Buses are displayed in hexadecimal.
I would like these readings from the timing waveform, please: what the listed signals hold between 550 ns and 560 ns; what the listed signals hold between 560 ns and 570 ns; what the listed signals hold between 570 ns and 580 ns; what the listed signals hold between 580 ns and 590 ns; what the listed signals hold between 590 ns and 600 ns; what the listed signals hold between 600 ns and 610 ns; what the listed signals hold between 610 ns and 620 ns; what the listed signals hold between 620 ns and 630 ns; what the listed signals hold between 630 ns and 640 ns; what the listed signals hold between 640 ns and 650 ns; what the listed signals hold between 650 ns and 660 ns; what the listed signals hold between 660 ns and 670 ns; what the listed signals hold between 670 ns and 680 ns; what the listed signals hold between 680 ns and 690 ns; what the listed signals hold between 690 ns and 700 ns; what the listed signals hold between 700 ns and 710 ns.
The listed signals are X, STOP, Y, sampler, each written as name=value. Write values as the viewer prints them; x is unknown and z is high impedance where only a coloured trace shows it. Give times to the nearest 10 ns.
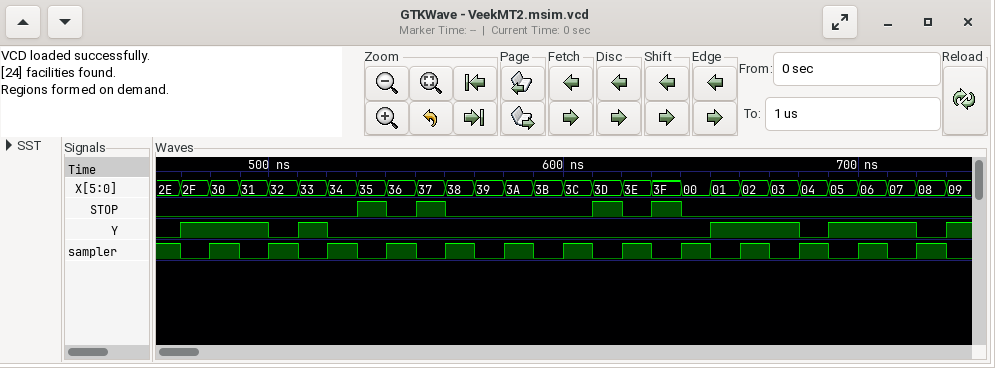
X=37, STOP=1, Y=0, sampler=0
X=38, STOP=0, Y=0, sampler=1
X=39, STOP=0, Y=0, sampler=0
X=3A, STOP=0, Y=0, sampler=1
X=3B, STOP=0, Y=0, sampler=0
X=3C, STOP=0, Y=0, sampler=1
X=3D, STOP=1, Y=0, sampler=0
X=3E, STOP=0, Y=0, sampler=1
X=3F, STOP=1, Y=0, sampler=0
X=00, STOP=0, Y=0, sampler=1
X=01, STOP=0, Y=1, sampler=0
X=02, STOP=0, Y=1, sampler=1
X=03, STOP=0, Y=1, sampler=0
X=04, STOP=0, Y=0, sampler=1
X=05, STOP=0, Y=1, sampler=0
X=06, STOP=0, Y=1, sampler=1
